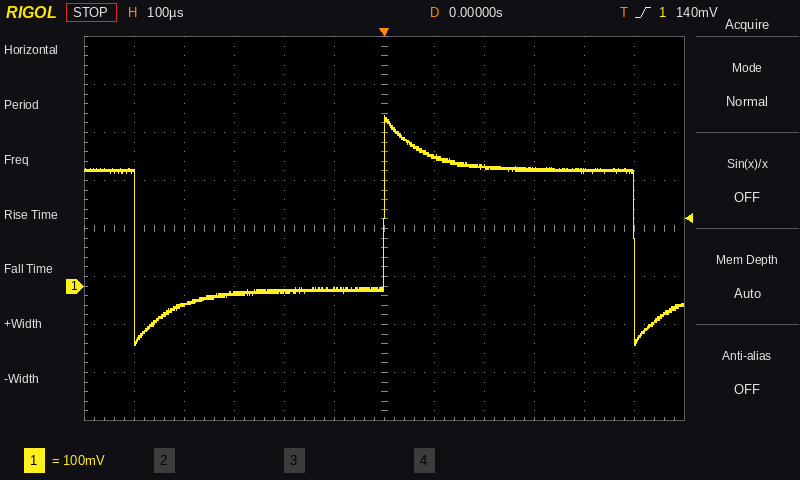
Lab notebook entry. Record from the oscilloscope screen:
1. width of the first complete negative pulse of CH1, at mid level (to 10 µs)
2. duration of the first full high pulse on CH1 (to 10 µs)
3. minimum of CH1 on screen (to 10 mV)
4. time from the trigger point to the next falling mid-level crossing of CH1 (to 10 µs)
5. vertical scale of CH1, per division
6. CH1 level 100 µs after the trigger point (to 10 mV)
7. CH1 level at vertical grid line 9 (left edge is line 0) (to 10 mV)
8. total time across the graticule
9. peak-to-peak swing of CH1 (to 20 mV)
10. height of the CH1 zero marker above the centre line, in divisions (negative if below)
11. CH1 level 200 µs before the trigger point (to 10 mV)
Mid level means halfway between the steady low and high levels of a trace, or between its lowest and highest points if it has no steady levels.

500 µs
500 µs
-120 mV
500 µs
100 mV
270 mV
240 mV
1.2 ms
480 mV
-1.2 div
-10 mV
